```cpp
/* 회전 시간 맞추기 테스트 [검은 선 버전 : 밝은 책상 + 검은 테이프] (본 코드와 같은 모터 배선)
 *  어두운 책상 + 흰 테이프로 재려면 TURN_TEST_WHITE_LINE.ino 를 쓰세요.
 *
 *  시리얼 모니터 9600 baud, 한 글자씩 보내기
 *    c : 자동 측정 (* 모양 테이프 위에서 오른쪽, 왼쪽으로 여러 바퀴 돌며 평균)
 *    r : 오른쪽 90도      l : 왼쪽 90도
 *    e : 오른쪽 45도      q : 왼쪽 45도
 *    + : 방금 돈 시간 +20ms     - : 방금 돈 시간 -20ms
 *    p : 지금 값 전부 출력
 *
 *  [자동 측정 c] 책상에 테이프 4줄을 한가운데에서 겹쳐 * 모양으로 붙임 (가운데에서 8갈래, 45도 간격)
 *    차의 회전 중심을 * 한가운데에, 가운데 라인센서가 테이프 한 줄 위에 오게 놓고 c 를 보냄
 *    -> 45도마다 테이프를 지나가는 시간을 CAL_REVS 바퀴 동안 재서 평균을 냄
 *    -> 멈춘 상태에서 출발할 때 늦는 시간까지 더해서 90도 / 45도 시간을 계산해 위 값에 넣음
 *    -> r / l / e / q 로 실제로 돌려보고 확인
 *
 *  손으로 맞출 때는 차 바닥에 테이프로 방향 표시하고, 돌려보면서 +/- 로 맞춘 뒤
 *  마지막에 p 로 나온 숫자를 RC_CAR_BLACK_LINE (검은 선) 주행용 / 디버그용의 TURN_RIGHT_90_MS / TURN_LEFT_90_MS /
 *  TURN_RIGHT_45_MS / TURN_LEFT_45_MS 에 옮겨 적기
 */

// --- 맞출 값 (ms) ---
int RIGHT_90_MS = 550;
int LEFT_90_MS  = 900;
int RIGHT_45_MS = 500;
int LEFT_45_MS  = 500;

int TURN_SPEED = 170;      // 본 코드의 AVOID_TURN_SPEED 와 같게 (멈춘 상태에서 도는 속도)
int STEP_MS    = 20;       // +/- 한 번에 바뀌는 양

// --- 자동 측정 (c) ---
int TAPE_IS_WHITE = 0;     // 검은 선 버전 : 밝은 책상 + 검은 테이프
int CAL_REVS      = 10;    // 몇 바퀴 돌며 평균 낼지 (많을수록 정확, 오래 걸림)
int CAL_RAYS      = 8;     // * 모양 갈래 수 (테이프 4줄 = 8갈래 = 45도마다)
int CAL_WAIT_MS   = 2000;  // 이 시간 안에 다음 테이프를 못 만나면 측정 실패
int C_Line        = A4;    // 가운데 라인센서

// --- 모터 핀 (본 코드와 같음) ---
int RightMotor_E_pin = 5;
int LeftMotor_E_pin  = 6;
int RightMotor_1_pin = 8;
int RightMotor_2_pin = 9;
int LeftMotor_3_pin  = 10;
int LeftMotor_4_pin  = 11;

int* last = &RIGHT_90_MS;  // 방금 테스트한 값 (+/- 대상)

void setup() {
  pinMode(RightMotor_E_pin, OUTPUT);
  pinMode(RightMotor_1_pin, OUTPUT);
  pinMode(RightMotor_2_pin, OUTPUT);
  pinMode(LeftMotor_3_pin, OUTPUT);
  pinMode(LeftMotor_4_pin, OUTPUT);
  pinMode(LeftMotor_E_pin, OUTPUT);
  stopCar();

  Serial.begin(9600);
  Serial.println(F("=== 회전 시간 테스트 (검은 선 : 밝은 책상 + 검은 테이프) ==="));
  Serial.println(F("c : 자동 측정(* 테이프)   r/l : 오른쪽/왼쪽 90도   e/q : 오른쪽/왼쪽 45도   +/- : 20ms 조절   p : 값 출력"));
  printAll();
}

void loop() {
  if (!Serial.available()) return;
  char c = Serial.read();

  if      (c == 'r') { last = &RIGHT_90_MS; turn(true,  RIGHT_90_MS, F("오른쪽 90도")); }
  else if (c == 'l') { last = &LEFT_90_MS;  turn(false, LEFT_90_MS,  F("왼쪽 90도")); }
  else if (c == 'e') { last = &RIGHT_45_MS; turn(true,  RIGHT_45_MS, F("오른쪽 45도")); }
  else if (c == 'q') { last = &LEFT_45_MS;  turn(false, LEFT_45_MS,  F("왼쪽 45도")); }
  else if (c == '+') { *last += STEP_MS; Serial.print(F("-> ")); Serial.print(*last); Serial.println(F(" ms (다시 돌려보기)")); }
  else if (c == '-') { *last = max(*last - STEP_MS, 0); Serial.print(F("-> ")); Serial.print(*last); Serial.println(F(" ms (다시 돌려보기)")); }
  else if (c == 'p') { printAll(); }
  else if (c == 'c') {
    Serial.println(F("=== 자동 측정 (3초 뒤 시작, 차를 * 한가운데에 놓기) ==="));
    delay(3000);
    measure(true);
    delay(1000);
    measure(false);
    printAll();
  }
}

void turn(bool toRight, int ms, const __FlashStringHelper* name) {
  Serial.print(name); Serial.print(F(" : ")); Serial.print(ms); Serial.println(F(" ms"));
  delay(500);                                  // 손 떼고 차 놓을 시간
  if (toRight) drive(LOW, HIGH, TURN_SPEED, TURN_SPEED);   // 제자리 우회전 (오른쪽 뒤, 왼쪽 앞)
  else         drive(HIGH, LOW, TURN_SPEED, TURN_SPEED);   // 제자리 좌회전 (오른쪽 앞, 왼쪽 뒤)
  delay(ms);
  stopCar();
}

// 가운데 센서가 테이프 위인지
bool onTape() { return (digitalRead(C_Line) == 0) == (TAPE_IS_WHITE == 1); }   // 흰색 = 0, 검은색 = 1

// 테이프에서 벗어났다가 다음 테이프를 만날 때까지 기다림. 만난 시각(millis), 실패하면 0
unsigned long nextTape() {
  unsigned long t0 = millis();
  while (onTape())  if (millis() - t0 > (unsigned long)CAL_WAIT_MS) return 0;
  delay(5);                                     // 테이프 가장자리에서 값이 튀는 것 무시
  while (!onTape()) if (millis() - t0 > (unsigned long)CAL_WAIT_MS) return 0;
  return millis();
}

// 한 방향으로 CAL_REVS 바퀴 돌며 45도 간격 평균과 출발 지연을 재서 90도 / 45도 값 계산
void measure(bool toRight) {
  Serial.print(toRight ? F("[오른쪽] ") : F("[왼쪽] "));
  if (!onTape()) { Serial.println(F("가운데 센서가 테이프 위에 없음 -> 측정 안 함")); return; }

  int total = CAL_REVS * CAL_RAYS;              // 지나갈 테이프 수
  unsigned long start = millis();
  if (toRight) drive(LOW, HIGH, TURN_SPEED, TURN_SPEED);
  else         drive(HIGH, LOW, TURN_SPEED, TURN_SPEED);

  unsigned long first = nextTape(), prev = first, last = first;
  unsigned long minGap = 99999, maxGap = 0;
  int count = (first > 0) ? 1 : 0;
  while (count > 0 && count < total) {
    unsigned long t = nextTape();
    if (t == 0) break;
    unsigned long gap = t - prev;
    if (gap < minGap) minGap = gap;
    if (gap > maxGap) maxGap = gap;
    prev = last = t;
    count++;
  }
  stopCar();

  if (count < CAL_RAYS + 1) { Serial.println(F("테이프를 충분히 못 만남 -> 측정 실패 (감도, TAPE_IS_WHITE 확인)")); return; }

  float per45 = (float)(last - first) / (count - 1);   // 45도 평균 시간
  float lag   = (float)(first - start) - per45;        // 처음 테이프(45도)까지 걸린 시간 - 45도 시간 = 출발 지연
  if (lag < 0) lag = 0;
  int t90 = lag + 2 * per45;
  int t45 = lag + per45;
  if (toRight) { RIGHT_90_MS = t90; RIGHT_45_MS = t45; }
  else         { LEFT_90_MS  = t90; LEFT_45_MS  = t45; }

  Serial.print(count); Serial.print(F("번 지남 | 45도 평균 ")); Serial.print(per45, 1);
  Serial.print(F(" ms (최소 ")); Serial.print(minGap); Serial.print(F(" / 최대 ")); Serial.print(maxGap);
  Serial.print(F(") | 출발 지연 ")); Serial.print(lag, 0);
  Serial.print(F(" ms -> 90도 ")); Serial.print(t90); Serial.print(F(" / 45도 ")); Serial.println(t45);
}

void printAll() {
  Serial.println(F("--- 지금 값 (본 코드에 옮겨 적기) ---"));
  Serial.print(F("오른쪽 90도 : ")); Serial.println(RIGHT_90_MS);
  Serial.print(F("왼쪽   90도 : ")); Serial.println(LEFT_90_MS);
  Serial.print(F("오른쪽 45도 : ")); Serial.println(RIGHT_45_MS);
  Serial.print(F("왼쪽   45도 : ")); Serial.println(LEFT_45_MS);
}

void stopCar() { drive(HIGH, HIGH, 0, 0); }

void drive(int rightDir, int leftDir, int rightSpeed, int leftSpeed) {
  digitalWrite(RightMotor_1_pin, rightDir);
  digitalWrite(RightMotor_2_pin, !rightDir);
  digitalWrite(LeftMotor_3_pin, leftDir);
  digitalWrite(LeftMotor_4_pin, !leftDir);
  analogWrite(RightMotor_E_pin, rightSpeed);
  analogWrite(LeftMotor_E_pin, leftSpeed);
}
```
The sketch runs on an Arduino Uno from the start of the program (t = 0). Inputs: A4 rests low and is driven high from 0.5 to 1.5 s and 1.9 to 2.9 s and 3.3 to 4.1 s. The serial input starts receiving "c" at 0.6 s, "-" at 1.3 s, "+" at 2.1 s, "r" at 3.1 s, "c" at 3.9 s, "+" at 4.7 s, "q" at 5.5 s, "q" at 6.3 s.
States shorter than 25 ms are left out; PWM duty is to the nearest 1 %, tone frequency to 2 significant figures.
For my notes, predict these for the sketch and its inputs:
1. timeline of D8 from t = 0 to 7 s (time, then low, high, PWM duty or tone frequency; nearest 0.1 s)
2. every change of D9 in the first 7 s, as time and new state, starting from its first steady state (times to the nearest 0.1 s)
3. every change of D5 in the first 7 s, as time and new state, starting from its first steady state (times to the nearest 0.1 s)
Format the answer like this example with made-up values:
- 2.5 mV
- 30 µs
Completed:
- 0 s high; 3.6 s low; 5.6 s high
- 0 s low; 3.6 s high; 5.6 s low
- 0 s low; 3.6 s PWM 67 %; 5.6 s low
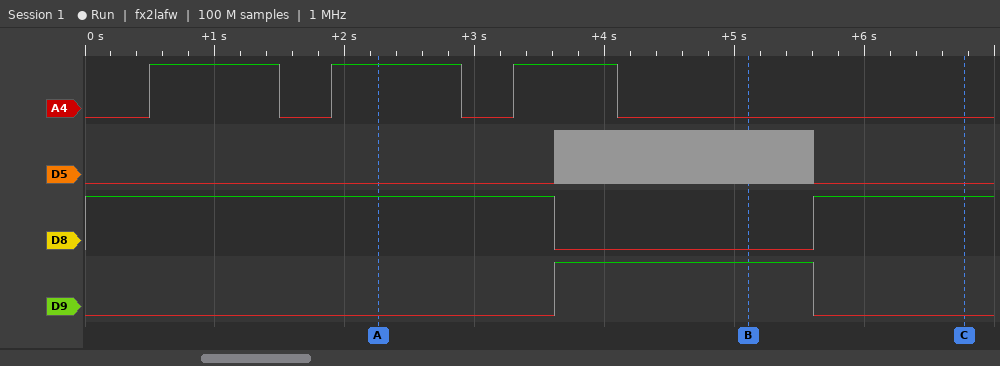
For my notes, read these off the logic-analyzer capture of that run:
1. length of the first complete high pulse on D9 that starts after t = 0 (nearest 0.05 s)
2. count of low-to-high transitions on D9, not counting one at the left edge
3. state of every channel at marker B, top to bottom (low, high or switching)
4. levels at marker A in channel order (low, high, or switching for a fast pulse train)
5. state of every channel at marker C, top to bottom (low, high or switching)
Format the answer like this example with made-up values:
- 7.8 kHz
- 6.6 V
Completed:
- 2.00 s
- 1
- A4 low, D5 switching, D8 low, D9 high
- A4 high, D5 low, D8 high, D9 low
- A4 low, D5 low, D8 high, D9 low
